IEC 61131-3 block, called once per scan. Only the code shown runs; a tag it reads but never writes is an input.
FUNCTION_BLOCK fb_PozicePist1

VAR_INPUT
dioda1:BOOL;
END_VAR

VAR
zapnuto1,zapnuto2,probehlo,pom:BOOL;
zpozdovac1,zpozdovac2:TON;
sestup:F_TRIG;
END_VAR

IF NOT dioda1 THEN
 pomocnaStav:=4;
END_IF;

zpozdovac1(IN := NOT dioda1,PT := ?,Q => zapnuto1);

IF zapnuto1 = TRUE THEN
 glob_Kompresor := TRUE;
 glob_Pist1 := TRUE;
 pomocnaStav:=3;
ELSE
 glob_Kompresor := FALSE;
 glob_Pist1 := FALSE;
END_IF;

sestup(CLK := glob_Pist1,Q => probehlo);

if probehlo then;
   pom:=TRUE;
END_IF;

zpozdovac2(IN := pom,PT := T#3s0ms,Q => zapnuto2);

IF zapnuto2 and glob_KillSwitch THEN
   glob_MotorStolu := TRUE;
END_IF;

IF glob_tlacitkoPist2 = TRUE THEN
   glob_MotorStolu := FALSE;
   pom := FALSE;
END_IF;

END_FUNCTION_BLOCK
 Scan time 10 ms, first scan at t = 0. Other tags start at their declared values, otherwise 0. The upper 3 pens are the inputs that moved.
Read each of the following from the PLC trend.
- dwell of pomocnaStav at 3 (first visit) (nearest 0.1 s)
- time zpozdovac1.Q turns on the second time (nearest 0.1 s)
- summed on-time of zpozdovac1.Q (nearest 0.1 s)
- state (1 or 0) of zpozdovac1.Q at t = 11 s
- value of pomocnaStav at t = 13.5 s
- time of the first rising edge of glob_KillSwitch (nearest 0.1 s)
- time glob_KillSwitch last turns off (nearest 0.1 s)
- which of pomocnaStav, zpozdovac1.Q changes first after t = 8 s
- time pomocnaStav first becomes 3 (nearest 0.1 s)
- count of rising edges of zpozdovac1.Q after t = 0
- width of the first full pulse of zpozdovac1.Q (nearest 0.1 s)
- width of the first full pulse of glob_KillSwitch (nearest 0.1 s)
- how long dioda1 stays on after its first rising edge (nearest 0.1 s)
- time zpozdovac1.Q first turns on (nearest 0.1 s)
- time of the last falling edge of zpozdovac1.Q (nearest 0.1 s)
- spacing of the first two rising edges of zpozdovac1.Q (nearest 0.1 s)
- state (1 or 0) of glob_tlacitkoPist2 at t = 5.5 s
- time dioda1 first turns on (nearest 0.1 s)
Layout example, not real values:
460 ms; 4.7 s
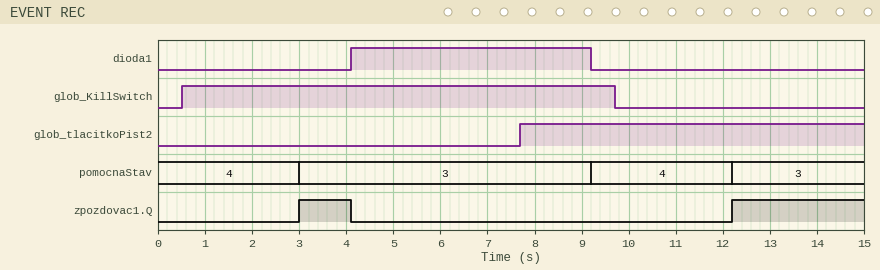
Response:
6.2 s; 12.2 s; 3.9 s; 0; 3; 0.5 s; 9.7 s; pomocnaStav; 3.0 s; 2; 1.1 s; 9.2 s; 5.1 s; 3.0 s; 4.1 s; 9.2 s; 0; 4.1 s
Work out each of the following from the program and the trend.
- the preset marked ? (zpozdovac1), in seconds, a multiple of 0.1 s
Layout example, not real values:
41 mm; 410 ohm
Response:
3.0 s
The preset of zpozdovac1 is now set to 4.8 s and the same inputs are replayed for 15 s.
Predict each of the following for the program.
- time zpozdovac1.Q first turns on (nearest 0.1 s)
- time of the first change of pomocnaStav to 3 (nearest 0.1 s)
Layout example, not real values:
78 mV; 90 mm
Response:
14.0 s; 14.0 s
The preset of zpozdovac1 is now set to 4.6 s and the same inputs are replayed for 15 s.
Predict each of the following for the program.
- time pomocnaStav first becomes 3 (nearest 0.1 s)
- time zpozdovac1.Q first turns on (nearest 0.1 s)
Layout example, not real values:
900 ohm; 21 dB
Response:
13.8 s; 13.8 s
